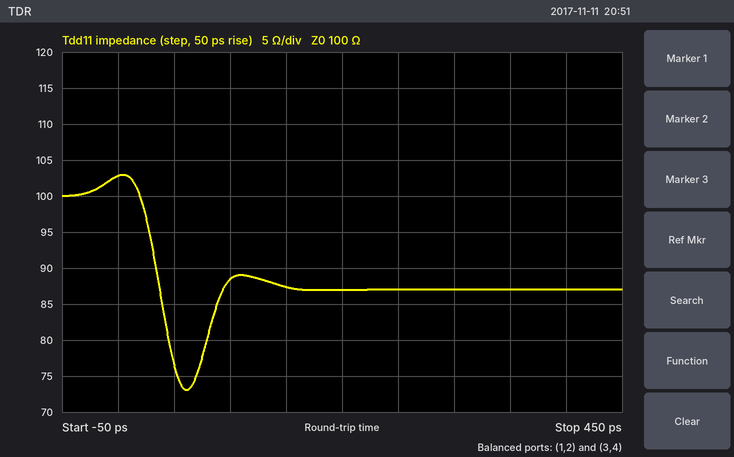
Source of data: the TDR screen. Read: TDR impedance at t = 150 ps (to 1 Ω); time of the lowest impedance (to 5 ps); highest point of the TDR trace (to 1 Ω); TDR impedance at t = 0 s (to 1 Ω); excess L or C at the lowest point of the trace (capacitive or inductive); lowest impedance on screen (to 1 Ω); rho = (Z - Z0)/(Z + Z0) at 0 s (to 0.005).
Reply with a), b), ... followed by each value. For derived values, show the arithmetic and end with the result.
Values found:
a) 87 Ω
b) 60 ps
c) 103 Ω
d) 103 Ω
e) capacitive
f) 73 Ω
g) (103 − 100)/(103 + 100) ≈ +0.015
